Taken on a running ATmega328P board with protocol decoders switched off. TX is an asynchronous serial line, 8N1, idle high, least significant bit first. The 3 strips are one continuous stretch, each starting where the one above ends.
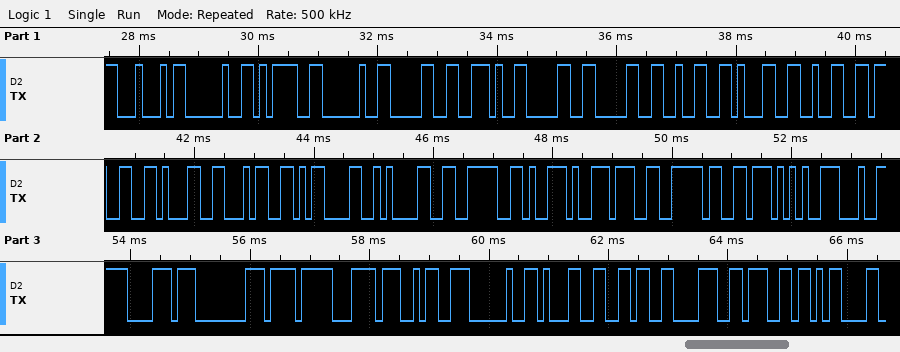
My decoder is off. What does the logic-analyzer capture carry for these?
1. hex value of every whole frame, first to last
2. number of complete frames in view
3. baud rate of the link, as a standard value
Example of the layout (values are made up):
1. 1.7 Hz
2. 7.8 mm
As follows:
1. 0x44 0x20 0x3D 0x20 0x30 0x2E 0x30 0x30 0x32 0x31 0x32 0x33 0x31 0x34 0x0D 0x0A 0xE6 0x96 0xB9 0xE6 0xB3 0x95 0xE4 0xB8 0x80 0xEF 0xBC 0x9A 0x20 0x31 0x36 0x38 0x67 0x0D
2. 34
3. 9600 baud
